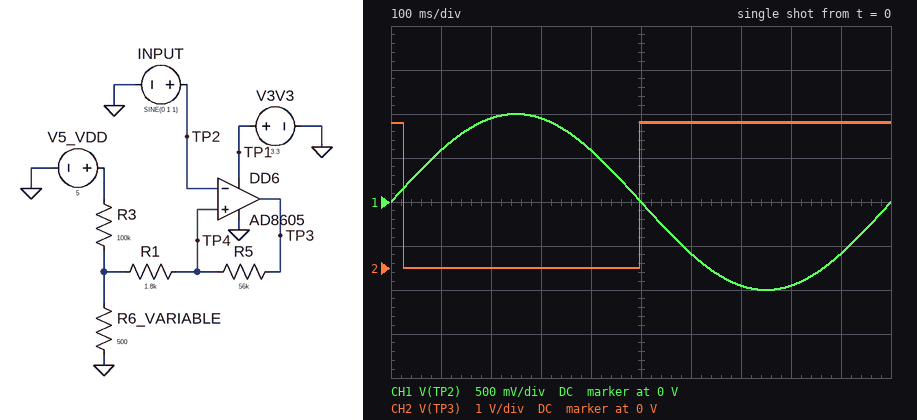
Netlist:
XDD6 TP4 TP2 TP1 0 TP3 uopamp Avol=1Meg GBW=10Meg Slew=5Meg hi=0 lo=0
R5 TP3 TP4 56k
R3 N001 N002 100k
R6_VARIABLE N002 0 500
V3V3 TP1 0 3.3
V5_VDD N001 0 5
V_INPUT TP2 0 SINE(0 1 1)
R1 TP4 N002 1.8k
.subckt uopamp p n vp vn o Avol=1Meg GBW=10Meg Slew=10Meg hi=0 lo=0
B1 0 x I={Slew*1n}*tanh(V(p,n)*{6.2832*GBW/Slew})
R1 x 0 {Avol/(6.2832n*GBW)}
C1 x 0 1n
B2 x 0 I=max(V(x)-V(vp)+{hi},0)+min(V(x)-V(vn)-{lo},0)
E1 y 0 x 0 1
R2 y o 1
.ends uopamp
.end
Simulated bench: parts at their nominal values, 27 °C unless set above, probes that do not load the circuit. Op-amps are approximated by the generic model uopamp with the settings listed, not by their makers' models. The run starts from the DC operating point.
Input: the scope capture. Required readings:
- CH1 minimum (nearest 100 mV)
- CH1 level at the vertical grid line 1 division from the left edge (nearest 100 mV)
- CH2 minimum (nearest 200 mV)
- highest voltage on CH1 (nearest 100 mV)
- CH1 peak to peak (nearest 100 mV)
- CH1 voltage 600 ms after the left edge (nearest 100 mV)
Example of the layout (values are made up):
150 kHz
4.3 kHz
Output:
-1.0 V
600 mV
0 V
1.0 V
2.0 V
-600 mV
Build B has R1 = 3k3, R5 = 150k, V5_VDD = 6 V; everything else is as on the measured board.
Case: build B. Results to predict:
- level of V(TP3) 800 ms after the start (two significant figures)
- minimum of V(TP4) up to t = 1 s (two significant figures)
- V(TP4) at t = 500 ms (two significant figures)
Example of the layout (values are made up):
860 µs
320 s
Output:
3.3 V
29 mV
110 mV
